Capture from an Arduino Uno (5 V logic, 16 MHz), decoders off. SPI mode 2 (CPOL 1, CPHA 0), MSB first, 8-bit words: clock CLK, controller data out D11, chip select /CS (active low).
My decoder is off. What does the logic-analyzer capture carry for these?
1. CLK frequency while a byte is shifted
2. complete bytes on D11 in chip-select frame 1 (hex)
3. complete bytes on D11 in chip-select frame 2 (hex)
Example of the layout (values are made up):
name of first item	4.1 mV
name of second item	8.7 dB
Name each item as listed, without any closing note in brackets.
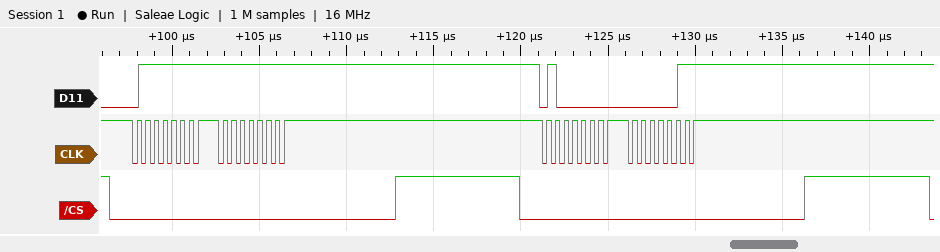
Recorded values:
CLK frequency while a byte is shifted	2 MHz
complete bytes on D11 in chip-select frame 1	7F FF
complete bytes on D11 in chip-select frame 2	40 03
